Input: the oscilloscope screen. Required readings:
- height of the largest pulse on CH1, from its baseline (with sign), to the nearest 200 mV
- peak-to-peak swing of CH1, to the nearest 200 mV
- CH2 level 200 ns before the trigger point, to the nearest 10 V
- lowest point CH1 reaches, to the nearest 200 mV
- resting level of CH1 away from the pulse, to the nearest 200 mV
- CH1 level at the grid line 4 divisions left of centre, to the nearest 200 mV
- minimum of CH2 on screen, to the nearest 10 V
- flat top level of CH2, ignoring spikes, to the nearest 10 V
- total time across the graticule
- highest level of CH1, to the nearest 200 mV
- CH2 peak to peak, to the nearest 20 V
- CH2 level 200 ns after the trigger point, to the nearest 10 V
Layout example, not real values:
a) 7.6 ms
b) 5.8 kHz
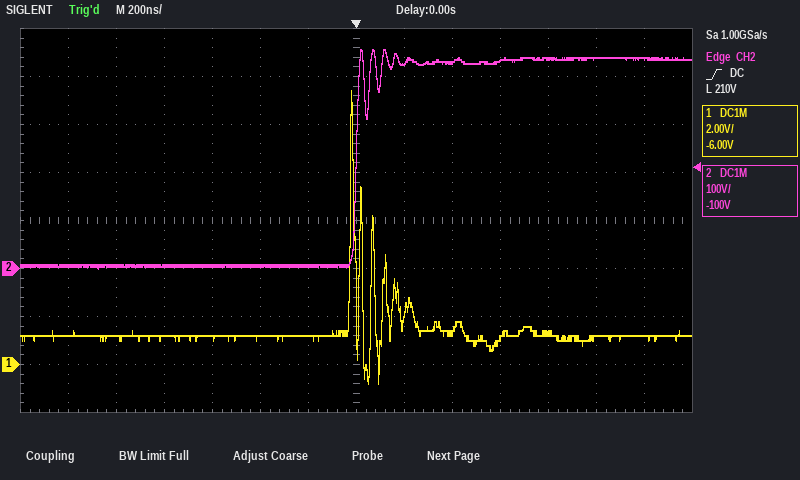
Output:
a) +10.2 V
b) 12.2 V
c) 10 V
d) -800 mV
e) 1.2 V
f) 1.2 V
g) 0 V
h) 440 V
i) 2.8 µs
j) 11.4 V
k) 460 V
l) 430 V
